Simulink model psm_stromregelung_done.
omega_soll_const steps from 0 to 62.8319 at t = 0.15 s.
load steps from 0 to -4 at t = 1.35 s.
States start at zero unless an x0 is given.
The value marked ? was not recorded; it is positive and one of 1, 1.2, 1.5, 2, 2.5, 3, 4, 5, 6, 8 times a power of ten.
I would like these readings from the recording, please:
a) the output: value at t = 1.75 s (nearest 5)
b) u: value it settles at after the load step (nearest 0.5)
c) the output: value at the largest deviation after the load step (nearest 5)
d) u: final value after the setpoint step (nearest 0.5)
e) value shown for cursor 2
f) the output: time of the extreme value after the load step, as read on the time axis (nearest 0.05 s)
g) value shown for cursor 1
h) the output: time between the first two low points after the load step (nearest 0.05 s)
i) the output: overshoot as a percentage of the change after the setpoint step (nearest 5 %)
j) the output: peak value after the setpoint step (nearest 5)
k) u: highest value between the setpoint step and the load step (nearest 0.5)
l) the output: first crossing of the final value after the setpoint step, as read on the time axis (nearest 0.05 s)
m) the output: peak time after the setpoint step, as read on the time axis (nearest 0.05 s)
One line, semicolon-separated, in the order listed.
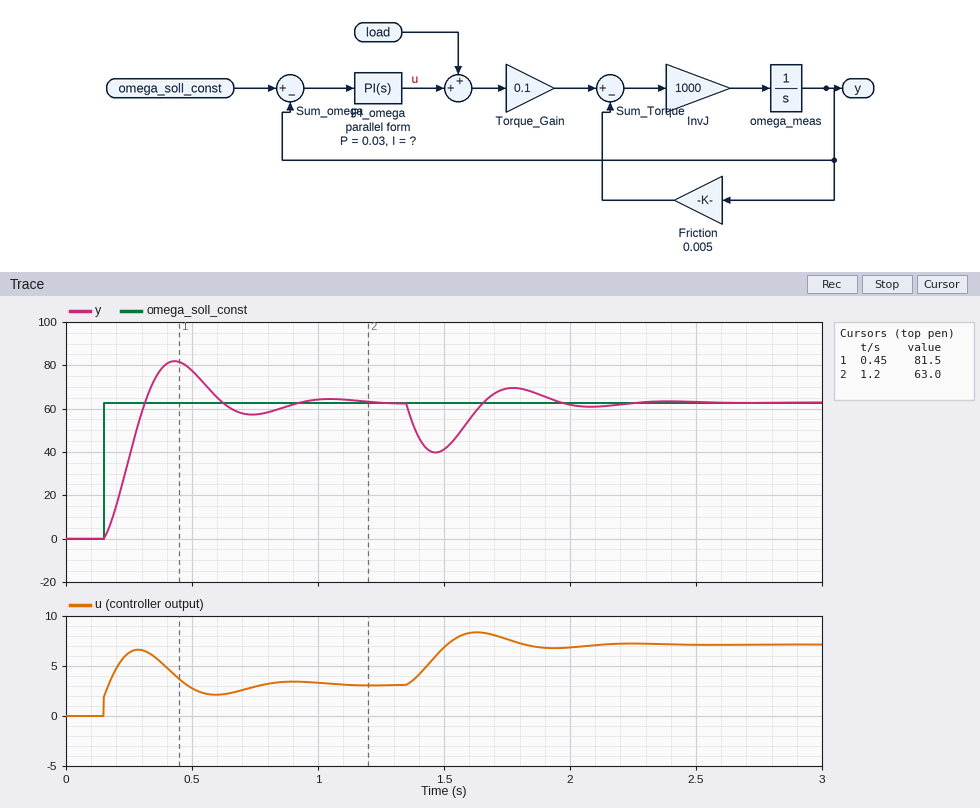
70; 7.0; 40; 3.0; 63.0; 1.45 s; 81.5; 0.60 s; 30 %; 80; 6.5; 0.30 s; 0.45 s
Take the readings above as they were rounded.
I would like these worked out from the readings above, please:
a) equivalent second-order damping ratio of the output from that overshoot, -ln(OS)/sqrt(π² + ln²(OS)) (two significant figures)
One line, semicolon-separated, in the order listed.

0.36
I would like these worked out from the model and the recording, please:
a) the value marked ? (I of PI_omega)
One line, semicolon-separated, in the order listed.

1.2
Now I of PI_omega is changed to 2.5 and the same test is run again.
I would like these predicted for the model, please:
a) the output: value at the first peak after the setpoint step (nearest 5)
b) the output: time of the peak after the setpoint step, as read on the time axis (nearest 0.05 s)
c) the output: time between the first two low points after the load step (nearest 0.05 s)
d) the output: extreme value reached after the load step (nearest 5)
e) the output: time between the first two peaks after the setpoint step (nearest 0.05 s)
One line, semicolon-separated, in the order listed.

90; 0.35 s; 0.40 s; 45; 0.40 s
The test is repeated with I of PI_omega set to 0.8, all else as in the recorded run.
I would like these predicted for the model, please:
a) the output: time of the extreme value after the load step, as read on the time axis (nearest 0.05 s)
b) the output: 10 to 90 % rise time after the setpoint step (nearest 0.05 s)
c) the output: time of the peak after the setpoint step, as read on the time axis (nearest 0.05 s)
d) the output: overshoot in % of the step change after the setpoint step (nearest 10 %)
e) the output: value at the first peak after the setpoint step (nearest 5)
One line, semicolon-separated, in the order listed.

1.50 s; 0.15 s; 0.50 s; 20 %; 75
